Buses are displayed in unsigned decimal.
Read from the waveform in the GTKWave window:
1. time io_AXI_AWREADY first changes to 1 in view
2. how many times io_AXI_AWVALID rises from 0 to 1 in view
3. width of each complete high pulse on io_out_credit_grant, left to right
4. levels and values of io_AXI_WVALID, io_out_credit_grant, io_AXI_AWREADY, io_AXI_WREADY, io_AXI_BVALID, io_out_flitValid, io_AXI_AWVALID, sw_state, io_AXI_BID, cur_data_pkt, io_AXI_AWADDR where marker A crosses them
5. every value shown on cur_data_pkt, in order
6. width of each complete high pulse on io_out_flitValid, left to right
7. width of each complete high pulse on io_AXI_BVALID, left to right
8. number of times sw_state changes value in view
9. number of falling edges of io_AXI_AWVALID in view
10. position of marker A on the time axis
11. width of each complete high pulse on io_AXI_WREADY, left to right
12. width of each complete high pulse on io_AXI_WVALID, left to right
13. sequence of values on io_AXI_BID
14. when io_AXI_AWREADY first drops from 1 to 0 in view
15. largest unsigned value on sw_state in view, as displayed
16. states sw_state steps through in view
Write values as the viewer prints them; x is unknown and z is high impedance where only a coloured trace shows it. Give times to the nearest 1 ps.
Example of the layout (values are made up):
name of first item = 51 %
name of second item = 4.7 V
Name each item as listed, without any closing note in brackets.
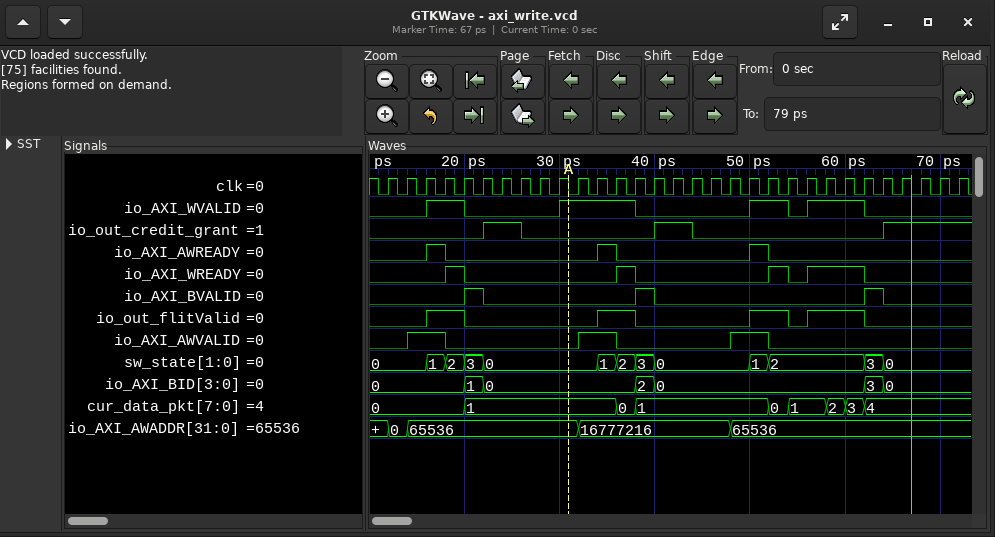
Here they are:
time io_AXI_AWREADY first changes to 1 in view = 16 ps
how many times io_AXI_AWVALID rises from 0 to 1 in view = 3
width of each complete high pulse on io_out_credit_grant, left to right = 4 ps, 4 ps
levels and values of io_AXI_WVALID, io_out_credit_grant, io_AXI_AWREADY, io_AXI_WREADY, io_AXI_BVALID, io_out_flitValid, io_AXI_AWVALID, sw_state, io_AXI_BID, cur_data_pkt, io_AXI_AWADDR where marker A crosses them = io_AXI_WVALID=1, io_out_credit_grant=0, io_AXI_AWREADY=0, io_AXI_WREADY=0, io_AXI_BVALID=0, io_out_flitValid=0, io_AXI_AWVALID=0, sw_state=0, io_AXI_BID=0, cur_data_pkt=1, io_AXI_AWADDR=65536
every value shown on cur_data_pkt, in order = 0, 1, 0, 1, 0, 1, 2, 3, 4
width of each complete high pulse on io_out_flitValid, left to right = 4 ps, 4 ps, 4 ps, 6 ps
width of each complete high pulse on io_AXI_BVALID, left to right = 2 ps, 2 ps, 2 ps
number of times sw_state changes value in view = 12
number of falling edges of io_AXI_AWVALID in view = 3
position of marker A on the time axis = 31 ps
width of each complete high pulse on io_AXI_WREADY, left to right = 2 ps, 2 ps, 2 ps, 6 ps
width of each complete high pulse on io_AXI_WVALID, left to right = 4 ps, 8 ps, 4 ps, 6 ps
sequence of values on io_AXI_BID = 0, 1, 0, 2, 0, 3, 0
when io_AXI_AWREADY first drops from 1 to 0 in view = 18 ps
largest unsigned value on sw_state in view, as displayed = 3
states sw_state steps through in view = 0, 1, 2, 3, 0, 1, 2, 3, 0, 1, 2, 3, 0
